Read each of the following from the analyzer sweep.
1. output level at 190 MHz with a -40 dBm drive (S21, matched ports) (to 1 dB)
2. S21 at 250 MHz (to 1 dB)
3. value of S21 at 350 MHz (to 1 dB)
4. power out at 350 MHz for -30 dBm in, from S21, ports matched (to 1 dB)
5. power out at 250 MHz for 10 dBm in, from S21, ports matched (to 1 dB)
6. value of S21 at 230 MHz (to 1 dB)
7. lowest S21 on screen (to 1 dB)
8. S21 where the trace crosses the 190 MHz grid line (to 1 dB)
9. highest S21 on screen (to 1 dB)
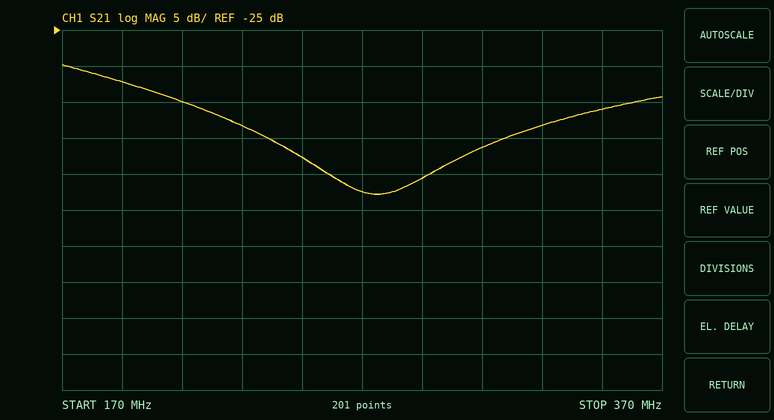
-72 dBm
-43 dB
-36 dB
-66 dBm
-33 dBm
-38 dB
-48 dB
-32 dB
-30 dB
